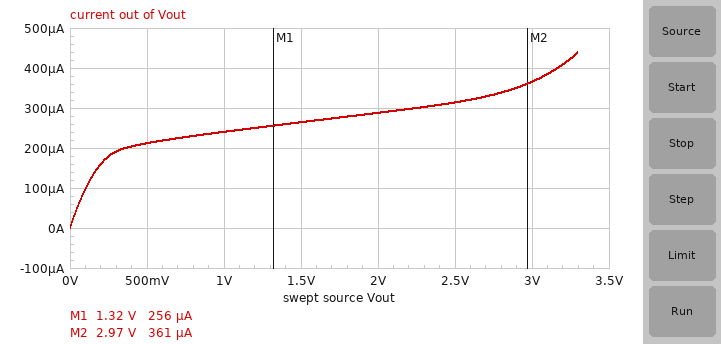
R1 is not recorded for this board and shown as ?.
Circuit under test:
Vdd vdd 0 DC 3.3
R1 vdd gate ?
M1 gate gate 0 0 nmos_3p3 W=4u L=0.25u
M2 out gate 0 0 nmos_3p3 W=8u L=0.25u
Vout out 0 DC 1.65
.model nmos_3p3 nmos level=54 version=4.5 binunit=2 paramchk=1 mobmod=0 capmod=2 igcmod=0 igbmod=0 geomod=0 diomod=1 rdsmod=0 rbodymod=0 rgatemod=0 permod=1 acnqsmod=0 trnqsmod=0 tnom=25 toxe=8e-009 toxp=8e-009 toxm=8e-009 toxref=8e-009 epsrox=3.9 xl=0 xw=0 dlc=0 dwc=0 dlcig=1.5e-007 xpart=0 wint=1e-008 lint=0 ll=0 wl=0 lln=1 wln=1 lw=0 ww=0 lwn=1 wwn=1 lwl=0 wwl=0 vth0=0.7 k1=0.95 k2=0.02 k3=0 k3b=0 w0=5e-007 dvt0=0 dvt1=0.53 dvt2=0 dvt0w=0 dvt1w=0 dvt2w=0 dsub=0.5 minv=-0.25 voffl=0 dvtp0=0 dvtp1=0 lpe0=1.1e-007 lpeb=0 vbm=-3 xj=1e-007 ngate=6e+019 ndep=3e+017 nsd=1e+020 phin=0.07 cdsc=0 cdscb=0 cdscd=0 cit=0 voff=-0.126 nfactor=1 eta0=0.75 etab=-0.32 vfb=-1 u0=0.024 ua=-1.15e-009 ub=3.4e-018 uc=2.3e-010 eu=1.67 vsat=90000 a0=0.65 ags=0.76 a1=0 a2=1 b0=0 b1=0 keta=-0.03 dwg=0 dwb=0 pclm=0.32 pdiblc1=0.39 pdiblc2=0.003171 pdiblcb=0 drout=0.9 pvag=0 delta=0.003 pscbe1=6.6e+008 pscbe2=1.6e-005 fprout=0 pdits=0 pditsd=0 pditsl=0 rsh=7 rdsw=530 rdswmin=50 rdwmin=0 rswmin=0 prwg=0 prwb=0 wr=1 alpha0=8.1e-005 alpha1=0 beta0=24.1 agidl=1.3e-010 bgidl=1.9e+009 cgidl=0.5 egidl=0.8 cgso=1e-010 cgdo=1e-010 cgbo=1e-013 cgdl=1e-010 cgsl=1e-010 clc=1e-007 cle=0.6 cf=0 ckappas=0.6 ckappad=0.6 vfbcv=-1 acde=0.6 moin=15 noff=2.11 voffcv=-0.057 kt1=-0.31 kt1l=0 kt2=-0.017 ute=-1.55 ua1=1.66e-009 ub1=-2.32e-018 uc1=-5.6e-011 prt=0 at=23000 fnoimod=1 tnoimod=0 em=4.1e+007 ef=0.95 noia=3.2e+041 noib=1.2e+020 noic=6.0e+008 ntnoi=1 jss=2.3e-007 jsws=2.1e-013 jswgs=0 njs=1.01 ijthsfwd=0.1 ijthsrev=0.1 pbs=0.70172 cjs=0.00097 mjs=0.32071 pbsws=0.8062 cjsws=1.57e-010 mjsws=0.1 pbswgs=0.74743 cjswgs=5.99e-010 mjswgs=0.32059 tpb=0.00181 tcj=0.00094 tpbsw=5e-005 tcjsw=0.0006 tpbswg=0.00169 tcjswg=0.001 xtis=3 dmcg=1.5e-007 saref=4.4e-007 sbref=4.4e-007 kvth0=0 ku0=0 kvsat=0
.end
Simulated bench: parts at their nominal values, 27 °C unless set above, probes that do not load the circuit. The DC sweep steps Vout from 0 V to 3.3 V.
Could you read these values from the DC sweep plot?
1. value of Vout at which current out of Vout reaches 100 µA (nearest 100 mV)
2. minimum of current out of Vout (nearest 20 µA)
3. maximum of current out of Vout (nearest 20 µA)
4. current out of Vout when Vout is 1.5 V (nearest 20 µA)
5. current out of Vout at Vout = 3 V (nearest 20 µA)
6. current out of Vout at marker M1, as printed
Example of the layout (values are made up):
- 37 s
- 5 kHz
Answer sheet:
- 100 mV
- 0 A
- 440 µA
- 260 µA
- 360 µA
- 256 µA
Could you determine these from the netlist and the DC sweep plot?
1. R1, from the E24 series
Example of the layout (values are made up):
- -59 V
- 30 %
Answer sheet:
- 16 kΩ
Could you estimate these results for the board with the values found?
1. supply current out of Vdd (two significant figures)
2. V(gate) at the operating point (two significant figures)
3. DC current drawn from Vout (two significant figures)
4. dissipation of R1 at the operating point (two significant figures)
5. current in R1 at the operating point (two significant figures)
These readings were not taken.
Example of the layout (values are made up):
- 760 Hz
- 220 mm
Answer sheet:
- 130 µA
- 1.3 V
- 270 µA
- 260 µW
- 130 µA
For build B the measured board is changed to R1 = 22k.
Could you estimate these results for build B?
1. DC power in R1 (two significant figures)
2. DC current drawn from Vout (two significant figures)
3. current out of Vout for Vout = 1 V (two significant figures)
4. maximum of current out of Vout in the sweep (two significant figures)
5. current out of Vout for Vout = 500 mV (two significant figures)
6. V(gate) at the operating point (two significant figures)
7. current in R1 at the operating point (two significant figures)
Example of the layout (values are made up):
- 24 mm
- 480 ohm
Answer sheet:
- 200 µW
- 210 µA
- 180 µA
- 360 µA
- 160 µA
- 1.2 V
- 95 µA
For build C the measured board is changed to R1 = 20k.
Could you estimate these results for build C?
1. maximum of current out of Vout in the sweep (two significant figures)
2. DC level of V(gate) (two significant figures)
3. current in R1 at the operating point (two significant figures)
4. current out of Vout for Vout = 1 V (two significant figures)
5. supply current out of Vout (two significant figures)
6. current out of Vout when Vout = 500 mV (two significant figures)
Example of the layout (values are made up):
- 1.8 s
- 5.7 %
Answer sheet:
- 380 µA
- 1.2 V
- 100 µA
- 200 µA
- 230 µA
- 170 µA
